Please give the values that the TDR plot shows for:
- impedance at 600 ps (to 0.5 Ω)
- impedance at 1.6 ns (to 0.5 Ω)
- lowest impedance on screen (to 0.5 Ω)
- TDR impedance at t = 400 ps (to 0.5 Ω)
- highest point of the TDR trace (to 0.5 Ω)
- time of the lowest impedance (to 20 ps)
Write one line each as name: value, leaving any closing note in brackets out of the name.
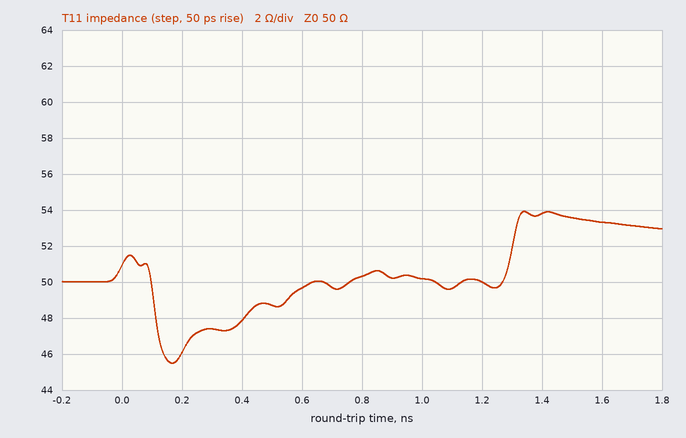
impedance at 600 ps: 49.5 Ω
impedance at 1.6 ns: 53.5 Ω
lowest impedance on screen: 45.5 Ω
TDR impedance at t = 400 ps: 48.0 Ω
highest point of the TDR trace: 54.0 Ω
time of the lowest impedance: 160 ps
